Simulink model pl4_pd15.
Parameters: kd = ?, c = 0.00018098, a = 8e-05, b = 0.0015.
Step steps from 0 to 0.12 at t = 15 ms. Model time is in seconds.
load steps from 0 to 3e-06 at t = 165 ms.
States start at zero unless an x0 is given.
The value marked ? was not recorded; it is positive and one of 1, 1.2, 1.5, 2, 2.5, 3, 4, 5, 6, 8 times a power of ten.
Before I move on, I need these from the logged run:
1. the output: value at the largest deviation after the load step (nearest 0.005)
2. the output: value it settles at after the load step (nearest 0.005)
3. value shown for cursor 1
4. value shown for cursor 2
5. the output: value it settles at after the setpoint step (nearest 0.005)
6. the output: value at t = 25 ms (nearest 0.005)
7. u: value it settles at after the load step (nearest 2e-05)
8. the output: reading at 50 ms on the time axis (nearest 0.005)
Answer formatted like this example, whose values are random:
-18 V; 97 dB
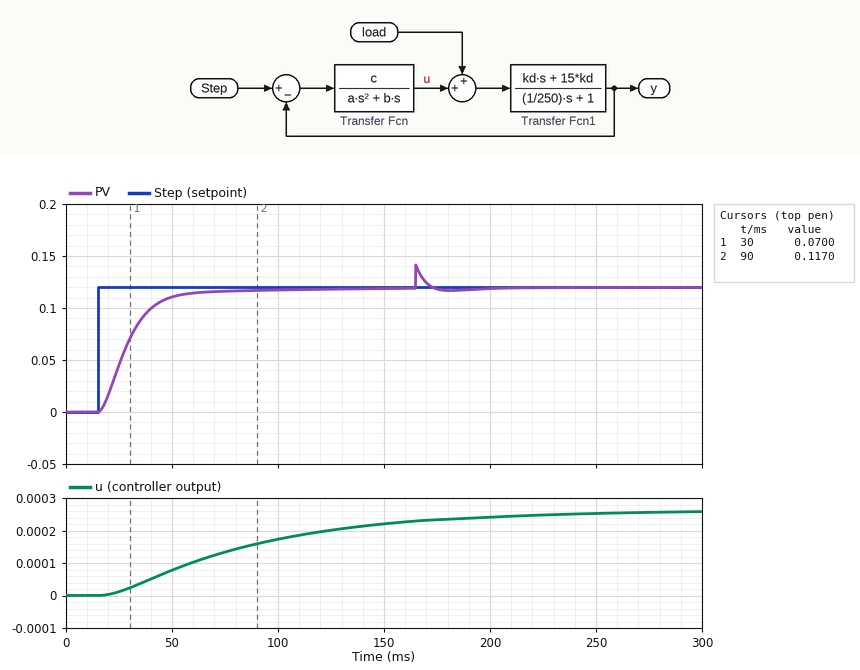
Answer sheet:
0.140; 0.120; 0.0700; 0.1170; 0.120; 0.045; 0.00026; 0.110
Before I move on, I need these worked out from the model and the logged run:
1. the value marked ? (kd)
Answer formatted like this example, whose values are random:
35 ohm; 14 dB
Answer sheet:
30
